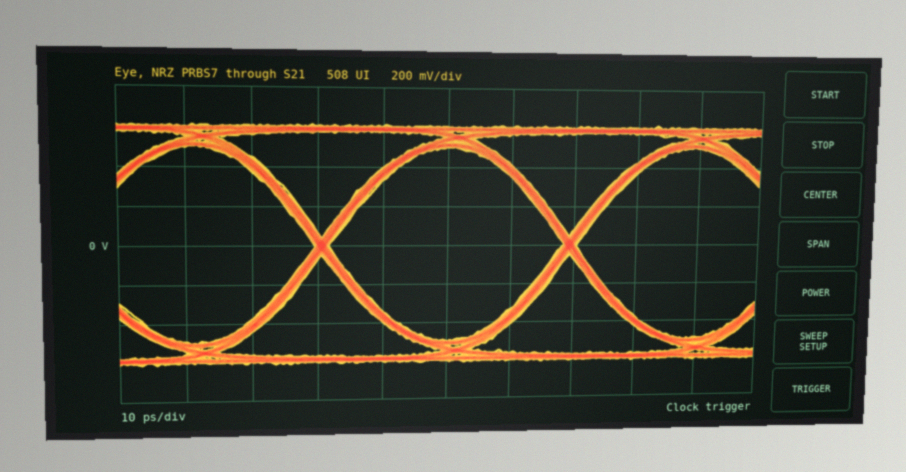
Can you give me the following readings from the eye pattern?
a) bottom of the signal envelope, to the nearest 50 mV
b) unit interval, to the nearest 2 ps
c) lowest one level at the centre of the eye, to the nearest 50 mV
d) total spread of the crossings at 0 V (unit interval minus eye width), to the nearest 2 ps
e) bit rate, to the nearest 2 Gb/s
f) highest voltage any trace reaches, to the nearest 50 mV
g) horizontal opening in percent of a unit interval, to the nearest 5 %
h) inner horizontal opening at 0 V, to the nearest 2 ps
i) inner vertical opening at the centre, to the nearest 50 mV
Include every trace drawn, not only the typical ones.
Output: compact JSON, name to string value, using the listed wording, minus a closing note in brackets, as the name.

{"bottom of the signal envelope, to the nearest 50 mV": "-600 mV", "unit interval, to the nearest 2 ps": "38 ps", "lowest one level at the centre of the eye, to the nearest 50 mV": "500 mV", "total spread of the crossings at 0 V (unit interval minus eye width), to the nearest 2 ps": "2 ps", "bit rate, to the nearest 2 Gb/s": "26 Gb/s", "highest voltage any trace reaches, to the nearest 50 mV": "600 mV", "horizontal opening in percent of a unit interval, to the nearest 5 %": "95 %", "inner horizontal opening at 0 V, to the nearest 2 ps": "36 ps", "inner vertical opening at the centre, to the nearest 50 mV": "1.00 V"}
